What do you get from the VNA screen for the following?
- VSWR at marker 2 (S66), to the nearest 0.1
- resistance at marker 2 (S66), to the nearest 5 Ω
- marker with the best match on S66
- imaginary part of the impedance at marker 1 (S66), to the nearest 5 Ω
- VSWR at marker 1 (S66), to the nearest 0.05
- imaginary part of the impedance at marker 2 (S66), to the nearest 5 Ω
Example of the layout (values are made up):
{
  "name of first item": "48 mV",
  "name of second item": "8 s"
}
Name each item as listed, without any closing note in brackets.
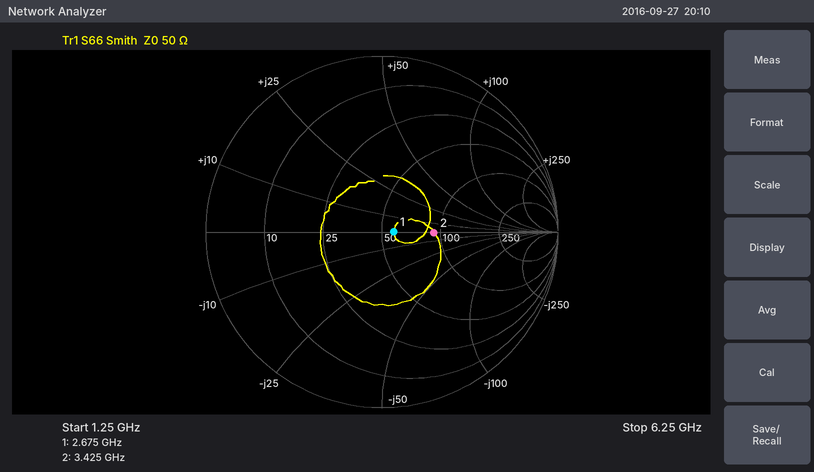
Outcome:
{
  "VSWR at marker 2 (S66), to the nearest 0.1": "1.8",
  "resistance at marker 2 (S66), to the nearest 5 Ω": "90 Ω",
  "marker with the best match on S66": "marker 1",
  "imaginary part of the impedance at marker 1 (S66), to the nearest 5 Ω": "0 Ω",
  "VSWR at marker 1 (S66), to the nearest 0.05": "1.15",
  "imaginary part of the impedance at marker 2 (S66), to the nearest 5 Ω": "0 Ω"
}
